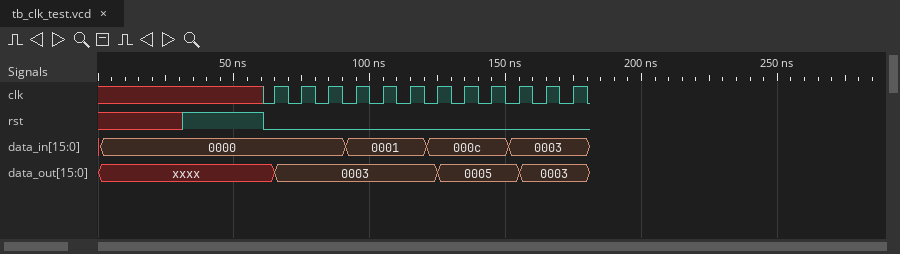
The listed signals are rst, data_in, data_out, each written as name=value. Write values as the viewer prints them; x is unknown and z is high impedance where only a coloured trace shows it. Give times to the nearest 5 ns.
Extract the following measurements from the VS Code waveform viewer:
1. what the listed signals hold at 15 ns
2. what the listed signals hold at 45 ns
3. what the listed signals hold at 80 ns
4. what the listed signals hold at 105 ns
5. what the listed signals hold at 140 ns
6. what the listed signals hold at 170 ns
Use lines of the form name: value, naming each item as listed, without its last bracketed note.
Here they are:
what the listed signals hold at 15 ns: rst=x, data_in=0000, data_out=xxxx
what the listed signals hold at 45 ns: rst=1, data_in=0000, data_out=xxxx
what the listed signals hold at 80 ns: rst=0, data_in=0000, data_out=0003
what the listed signals hold at 105 ns: rst=0, data_in=0001, data_out=0003
what the listed signals hold at 140 ns: rst=0, data_in=000c, data_out=0005
what the listed signals hold at 170 ns: rst=0, data_in=0003, data_out=0003
